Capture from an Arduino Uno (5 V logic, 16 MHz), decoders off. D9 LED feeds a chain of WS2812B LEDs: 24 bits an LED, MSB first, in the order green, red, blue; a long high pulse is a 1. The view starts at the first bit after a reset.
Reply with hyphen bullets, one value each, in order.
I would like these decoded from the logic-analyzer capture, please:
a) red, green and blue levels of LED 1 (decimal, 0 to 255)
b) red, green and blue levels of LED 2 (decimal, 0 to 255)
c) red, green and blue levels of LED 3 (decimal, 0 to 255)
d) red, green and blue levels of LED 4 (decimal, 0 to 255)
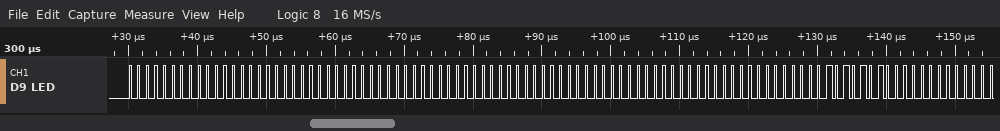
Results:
- 0, 0, 0
- 0, 0, 0
- 0, 0, 0
- 85, 0, 0
